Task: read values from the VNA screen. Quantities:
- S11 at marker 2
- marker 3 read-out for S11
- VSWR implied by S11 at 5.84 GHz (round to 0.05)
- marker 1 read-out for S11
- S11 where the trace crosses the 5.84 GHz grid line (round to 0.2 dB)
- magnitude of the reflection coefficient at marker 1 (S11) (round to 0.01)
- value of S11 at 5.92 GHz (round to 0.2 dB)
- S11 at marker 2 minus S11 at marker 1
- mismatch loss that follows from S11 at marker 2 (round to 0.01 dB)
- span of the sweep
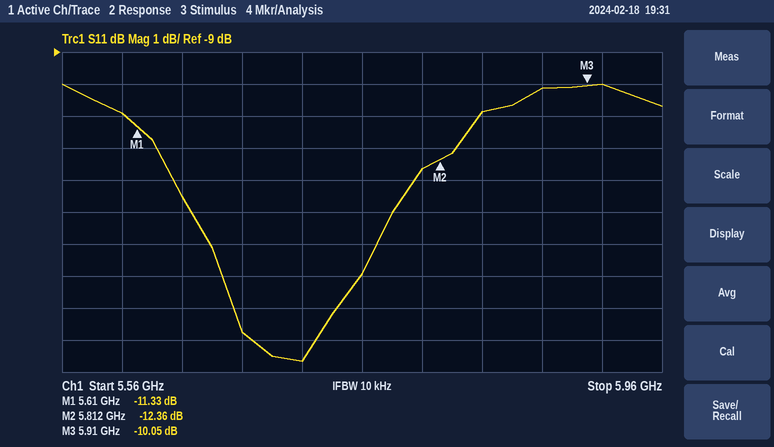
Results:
-12.36 dB
-10.05 dB
1.80
-11.33 dB
-10.8 dB
0.27
-10.0 dB
-1.03 dB
0.26 dB
400 MHz
